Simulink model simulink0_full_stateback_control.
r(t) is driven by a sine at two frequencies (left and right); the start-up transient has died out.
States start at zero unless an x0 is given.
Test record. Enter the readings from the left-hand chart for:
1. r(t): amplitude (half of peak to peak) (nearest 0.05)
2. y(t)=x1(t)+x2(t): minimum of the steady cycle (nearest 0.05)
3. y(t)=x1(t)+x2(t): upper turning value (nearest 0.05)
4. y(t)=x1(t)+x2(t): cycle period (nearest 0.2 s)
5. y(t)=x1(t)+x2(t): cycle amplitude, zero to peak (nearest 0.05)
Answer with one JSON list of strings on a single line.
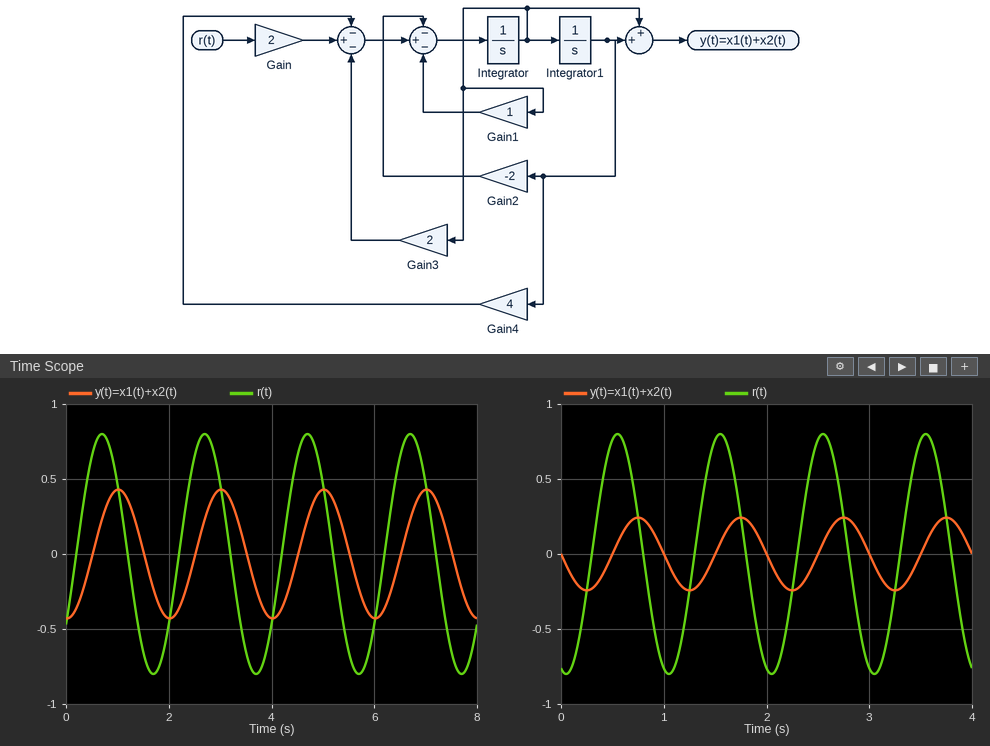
["0.80", "-0.45", "0.45", "2.0 s", "0.45"]
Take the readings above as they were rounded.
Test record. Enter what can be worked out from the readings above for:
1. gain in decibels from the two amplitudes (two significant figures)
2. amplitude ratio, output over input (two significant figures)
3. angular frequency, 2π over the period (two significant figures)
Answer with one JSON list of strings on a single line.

["-5.0 dB", "0.56", "3.1 rad/s"]
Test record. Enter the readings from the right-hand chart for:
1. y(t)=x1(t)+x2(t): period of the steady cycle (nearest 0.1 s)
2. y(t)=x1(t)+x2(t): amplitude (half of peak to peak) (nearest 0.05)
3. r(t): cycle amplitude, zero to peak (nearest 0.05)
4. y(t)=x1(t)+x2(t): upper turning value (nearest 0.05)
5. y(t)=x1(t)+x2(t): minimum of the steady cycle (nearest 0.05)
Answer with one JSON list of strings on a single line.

["1.0 s", "0.25", "0.80", "0.25", "-0.25"]
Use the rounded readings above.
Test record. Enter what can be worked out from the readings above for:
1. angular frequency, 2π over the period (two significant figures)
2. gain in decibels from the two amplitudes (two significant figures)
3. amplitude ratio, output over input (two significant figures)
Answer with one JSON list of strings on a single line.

["6.3 rad/s", "-10 dB", "0.31"]
